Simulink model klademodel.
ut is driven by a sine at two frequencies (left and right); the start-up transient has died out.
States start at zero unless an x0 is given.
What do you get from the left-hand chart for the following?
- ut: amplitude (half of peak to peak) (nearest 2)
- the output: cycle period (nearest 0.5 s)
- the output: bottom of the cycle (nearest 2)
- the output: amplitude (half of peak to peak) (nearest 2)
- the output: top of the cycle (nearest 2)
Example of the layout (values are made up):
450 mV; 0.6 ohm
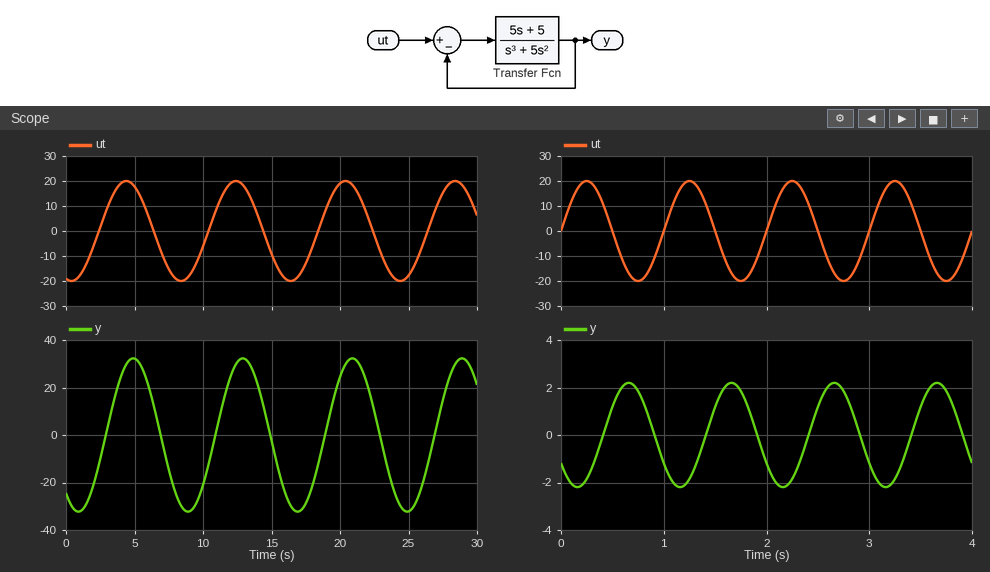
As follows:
20; 8.0 s; -32; 32; 32
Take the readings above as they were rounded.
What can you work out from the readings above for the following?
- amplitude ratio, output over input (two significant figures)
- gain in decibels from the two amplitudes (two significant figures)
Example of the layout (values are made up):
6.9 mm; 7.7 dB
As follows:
1.6; 4.1 dB
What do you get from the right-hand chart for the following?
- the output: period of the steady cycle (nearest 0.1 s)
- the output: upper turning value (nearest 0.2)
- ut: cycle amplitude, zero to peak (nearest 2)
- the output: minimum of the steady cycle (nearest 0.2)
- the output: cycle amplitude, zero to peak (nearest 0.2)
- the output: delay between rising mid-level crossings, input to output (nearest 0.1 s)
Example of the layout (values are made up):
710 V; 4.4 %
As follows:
1.0 s; 2.2; 20; -2.2; 2.2; 0.4 s
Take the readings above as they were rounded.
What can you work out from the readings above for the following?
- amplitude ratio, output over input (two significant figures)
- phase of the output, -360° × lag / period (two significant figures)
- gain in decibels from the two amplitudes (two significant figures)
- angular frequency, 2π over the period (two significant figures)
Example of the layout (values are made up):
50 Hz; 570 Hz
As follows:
0.11; -140°; -19 dB; 6.3 rad/s
